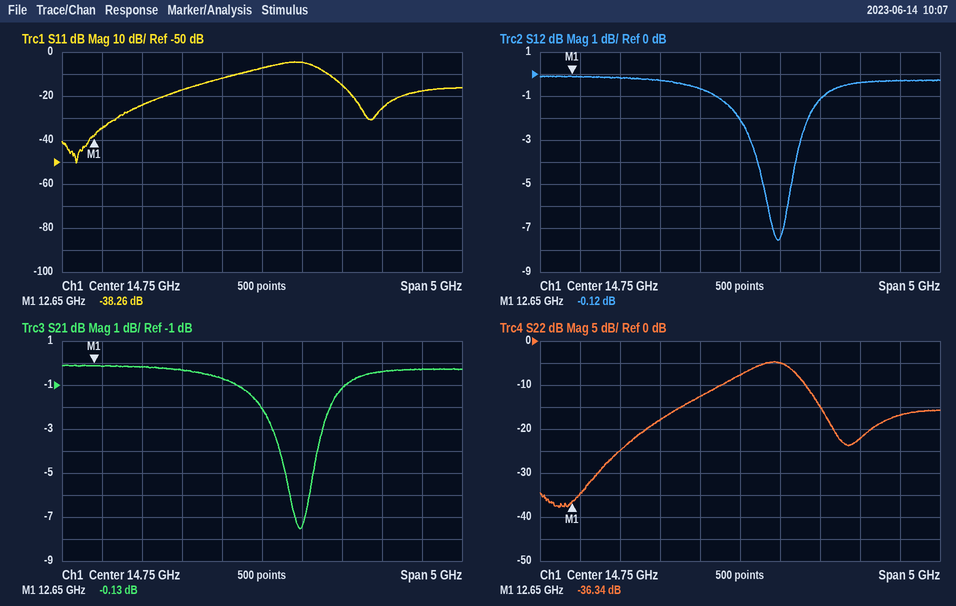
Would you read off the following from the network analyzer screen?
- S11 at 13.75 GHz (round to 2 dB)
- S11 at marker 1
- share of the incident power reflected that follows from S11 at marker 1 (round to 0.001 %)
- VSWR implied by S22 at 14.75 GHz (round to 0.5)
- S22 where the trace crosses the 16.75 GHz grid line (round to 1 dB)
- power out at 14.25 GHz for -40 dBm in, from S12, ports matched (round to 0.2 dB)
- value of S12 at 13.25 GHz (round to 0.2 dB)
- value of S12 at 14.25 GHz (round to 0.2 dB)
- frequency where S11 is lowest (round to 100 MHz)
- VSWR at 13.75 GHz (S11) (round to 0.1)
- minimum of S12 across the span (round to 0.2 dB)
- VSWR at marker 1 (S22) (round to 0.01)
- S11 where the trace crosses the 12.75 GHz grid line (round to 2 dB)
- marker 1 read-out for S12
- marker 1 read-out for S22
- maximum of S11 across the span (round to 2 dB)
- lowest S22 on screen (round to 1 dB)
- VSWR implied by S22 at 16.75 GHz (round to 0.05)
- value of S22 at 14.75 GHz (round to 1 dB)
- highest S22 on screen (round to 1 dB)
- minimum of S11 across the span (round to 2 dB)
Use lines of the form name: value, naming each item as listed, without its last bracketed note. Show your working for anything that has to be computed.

S11 at 13.75 GHz: -18 dB
S11 at marker 1: -38.26 dB
share of the incident power reflected that follows from S11 at marker 1: 10^(-38.26/10) ≈ 0.015 %
VSWR implied by S22 at 14.75 GHz: |Γ| = 10^(-8/20) = 0.3981; VSWR = (1 + 0.3981)/(1 − 0.3981) ≈ 2.32, so 2.5 to the nearest 0.5
S22 where the trace crosses the 16.75 GHz grid line: -17 dB
power out at 14.25 GHz for -40 dBm in, from S12, ports matched: -40 dBm + (-0.6 dB) = -40.6 dBm
value of S12 at 13.25 GHz: -0.2 dB
value of S12 at 14.25 GHz: -0.6 dB
frequency where S11 is lowest: 12.4 GHz
VSWR at 13.75 GHz (S11): |Γ| = 10^(-18/20) = 0.1259; VSWR = (1 + 0.1259)/(1 − 0.1259) ≈ 1.3
minimum of S12 across the span: -7.6 dB
VSWR at marker 1 (S22): (1 + 0.0152)/(1 − 0.0152) ≈ 1.03
S11 where the trace crosses the 12.75 GHz grid line: -34 dB
marker 1 read-out for S12: -0.12 dB
marker 1 read-out for S22: -36.34 dB
maximum of S11 across the span: -4 dB
lowest S22 on screen: -38 dB
VSWR implied by S22 at 16.75 GHz: |Γ| = 10^(-17/20) = 0.1413; VSWR = (1 + 0.1413)/(1 − 0.1413) ≈ 1.33, so 1.35 to the nearest 0.05
value of S22 at 14.75 GHz: -8 dB
highest S22 on screen: -5 dB
minimum of S11 across the span: -50 dB
